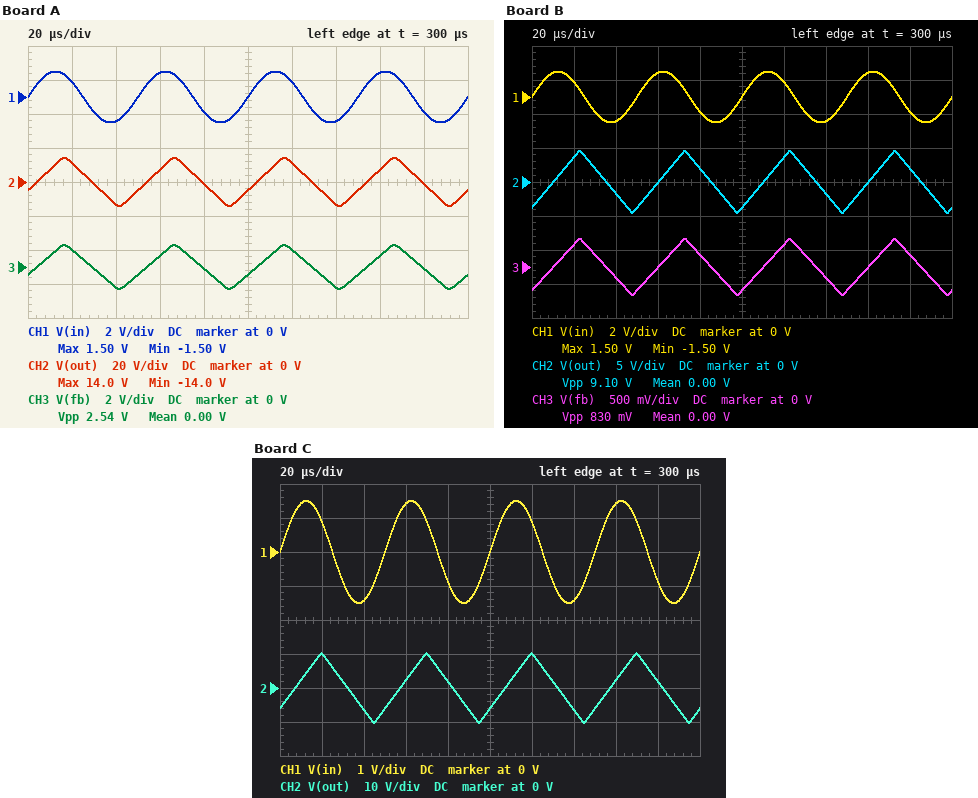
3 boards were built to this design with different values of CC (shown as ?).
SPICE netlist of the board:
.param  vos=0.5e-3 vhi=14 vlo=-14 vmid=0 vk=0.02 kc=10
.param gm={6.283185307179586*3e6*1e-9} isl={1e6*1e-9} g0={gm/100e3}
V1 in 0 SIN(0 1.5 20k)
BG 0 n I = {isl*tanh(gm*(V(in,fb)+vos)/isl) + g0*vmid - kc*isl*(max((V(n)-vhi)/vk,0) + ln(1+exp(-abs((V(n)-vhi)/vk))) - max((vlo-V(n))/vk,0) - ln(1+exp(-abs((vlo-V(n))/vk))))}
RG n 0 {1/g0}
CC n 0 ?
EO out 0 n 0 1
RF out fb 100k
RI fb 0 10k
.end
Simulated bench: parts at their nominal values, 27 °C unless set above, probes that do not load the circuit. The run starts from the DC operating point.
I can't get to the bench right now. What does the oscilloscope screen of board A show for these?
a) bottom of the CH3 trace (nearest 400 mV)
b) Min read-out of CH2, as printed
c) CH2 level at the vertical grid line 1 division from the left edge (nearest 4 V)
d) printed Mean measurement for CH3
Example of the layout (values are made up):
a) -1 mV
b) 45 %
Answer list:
a) -1.2 V
b) -14.0 V
c) 12 V
d) 0.00 V
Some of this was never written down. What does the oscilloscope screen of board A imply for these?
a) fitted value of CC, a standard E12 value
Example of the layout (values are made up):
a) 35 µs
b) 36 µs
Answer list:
a) 820 pF
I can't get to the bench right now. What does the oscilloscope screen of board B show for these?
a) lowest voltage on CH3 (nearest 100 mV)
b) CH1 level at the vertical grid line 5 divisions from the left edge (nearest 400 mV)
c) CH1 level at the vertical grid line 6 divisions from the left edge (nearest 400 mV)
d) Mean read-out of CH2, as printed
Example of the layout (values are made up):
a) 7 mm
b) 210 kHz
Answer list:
a) -400 mV
b) 0 V
c) 800 mV
d) 0.00 V
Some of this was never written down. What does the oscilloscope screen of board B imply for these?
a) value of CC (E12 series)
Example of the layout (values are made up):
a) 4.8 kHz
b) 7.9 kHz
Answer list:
a) 2.7 nF
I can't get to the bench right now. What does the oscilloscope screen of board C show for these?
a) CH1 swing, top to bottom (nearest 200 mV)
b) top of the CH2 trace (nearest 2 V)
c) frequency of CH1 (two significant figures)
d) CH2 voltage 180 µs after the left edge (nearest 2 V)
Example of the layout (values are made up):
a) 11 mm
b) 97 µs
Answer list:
a) 3.0 V
b) 10 V
c) 20 kHz
d) 2 V
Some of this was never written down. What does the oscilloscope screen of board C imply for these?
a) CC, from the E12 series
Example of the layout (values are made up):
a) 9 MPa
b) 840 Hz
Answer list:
a) 1.2 nF
